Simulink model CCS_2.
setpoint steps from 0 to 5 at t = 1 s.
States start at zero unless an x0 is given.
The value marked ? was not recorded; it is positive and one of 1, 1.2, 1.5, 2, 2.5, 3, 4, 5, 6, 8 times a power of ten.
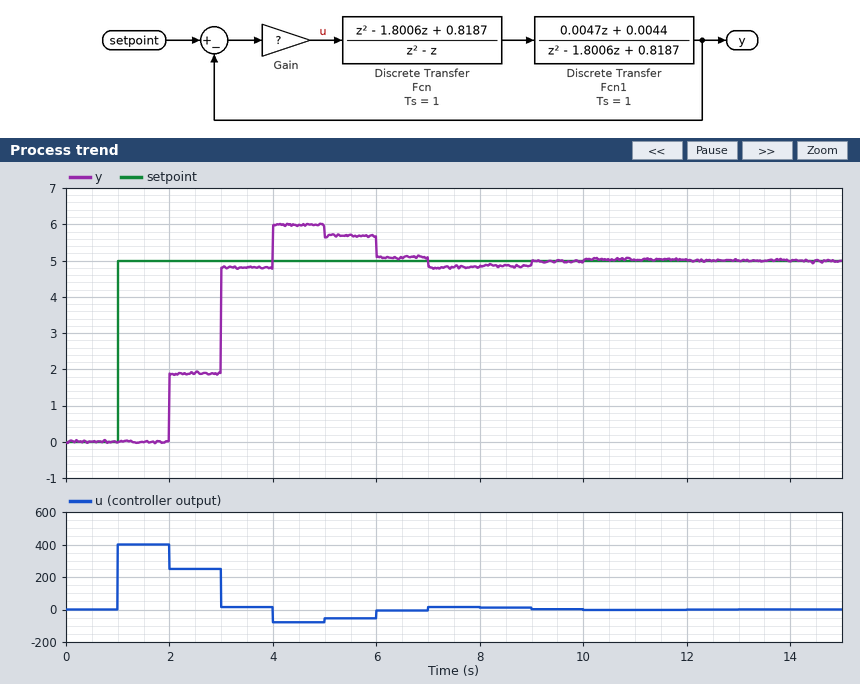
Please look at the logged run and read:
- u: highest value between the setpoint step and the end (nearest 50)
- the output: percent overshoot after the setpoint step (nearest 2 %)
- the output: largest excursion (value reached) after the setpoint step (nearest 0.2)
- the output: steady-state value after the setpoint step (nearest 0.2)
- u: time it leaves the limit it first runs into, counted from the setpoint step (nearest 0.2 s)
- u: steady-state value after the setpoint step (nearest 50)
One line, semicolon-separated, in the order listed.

400; 20 %; 6.0; 5.0; 1.0 s; 0
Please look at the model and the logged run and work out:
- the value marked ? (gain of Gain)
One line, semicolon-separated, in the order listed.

80
